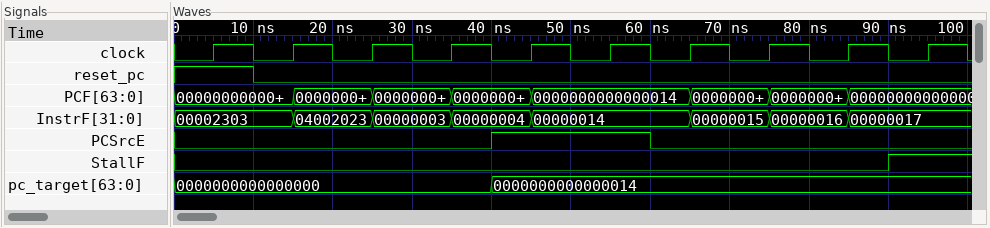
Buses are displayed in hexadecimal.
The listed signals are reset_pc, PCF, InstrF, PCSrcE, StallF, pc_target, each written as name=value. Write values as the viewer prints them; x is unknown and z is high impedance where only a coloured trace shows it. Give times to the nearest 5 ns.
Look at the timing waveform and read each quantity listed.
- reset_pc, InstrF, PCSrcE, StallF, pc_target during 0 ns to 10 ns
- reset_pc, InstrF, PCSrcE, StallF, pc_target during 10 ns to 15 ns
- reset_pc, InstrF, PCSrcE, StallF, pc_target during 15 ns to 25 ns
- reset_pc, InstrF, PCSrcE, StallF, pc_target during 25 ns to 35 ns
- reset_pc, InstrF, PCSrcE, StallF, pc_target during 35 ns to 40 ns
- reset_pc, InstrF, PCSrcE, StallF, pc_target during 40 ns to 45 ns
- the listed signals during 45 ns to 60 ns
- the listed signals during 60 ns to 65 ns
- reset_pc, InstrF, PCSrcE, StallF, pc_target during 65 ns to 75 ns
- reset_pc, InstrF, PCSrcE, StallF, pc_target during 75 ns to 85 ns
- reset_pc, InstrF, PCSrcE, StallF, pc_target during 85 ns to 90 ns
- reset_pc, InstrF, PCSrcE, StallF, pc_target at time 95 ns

reset_pc=1, InstrF=00002303, PCSrcE=0, StallF=0, pc_target=0000000000000000
reset_pc=0, InstrF=00002303, PCSrcE=0, StallF=0, pc_target=0000000000000000
reset_pc=0, InstrF=04002023, PCSrcE=0, StallF=0, pc_target=0000000000000000
reset_pc=0, InstrF=00000003, PCSrcE=0, StallF=0, pc_target=0000000000000000
reset_pc=0, InstrF=00000004, PCSrcE=0, StallF=0, pc_target=0000000000000000
reset_pc=0, InstrF=00000004, PCSrcE=1, StallF=0, pc_target=0000000000000014
reset_pc=0, PCF=0000000000000014, InstrF=00000014, PCSrcE=1, StallF=0, pc_target=0000000000000014
reset_pc=0, PCF=0000000000000014, InstrF=00000014, PCSrcE=0, StallF=0, pc_target=0000000000000014
reset_pc=0, InstrF=00000015, PCSrcE=0, StallF=0, pc_target=0000000000000014
reset_pc=0, InstrF=00000016, PCSrcE=0, StallF=0, pc_target=0000000000000014
reset_pc=0, InstrF=00000017, PCSrcE=0, StallF=0, pc_target=0000000000000014
reset_pc=0, InstrF=00000017, PCSrcE=0, StallF=1, pc_target=0000000000000014
